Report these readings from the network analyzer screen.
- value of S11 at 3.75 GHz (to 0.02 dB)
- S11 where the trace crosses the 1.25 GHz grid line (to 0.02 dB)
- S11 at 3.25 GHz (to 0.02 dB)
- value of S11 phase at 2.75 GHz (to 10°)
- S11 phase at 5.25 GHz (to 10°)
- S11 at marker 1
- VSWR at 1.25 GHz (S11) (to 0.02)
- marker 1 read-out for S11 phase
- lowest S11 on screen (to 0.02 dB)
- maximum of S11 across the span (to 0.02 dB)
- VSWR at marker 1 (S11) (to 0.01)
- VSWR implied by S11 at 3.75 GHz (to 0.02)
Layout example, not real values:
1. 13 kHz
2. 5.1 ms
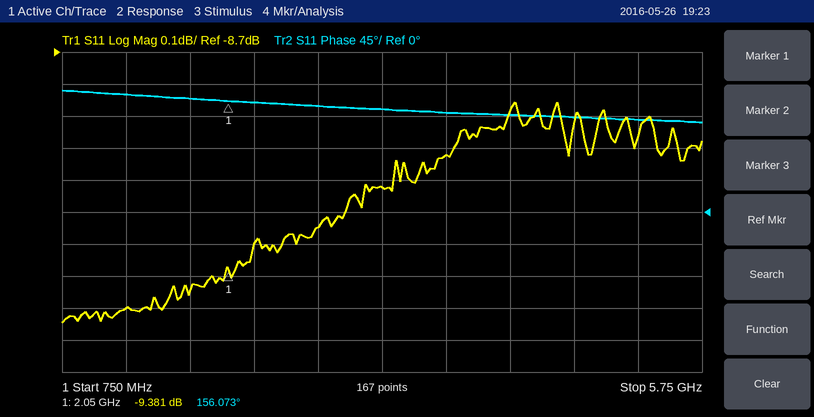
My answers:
1. -9.02 dB
2. -9.50 dB
3. -9.12 dB
4. 150°
5. 130°
6. -9.381 dB
7. 2.00
8. 156.073°
9. -9.54 dB
10. -8.86 dB
11. 2.03
12. 2.10
